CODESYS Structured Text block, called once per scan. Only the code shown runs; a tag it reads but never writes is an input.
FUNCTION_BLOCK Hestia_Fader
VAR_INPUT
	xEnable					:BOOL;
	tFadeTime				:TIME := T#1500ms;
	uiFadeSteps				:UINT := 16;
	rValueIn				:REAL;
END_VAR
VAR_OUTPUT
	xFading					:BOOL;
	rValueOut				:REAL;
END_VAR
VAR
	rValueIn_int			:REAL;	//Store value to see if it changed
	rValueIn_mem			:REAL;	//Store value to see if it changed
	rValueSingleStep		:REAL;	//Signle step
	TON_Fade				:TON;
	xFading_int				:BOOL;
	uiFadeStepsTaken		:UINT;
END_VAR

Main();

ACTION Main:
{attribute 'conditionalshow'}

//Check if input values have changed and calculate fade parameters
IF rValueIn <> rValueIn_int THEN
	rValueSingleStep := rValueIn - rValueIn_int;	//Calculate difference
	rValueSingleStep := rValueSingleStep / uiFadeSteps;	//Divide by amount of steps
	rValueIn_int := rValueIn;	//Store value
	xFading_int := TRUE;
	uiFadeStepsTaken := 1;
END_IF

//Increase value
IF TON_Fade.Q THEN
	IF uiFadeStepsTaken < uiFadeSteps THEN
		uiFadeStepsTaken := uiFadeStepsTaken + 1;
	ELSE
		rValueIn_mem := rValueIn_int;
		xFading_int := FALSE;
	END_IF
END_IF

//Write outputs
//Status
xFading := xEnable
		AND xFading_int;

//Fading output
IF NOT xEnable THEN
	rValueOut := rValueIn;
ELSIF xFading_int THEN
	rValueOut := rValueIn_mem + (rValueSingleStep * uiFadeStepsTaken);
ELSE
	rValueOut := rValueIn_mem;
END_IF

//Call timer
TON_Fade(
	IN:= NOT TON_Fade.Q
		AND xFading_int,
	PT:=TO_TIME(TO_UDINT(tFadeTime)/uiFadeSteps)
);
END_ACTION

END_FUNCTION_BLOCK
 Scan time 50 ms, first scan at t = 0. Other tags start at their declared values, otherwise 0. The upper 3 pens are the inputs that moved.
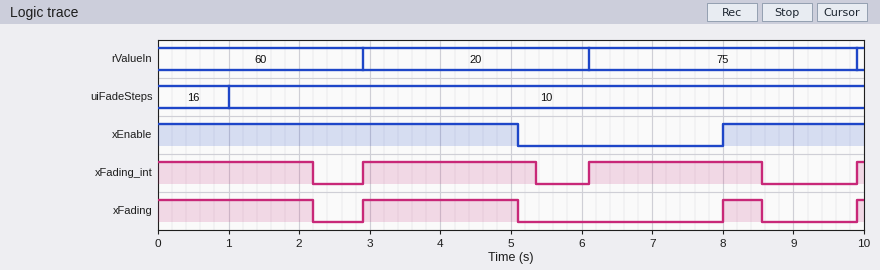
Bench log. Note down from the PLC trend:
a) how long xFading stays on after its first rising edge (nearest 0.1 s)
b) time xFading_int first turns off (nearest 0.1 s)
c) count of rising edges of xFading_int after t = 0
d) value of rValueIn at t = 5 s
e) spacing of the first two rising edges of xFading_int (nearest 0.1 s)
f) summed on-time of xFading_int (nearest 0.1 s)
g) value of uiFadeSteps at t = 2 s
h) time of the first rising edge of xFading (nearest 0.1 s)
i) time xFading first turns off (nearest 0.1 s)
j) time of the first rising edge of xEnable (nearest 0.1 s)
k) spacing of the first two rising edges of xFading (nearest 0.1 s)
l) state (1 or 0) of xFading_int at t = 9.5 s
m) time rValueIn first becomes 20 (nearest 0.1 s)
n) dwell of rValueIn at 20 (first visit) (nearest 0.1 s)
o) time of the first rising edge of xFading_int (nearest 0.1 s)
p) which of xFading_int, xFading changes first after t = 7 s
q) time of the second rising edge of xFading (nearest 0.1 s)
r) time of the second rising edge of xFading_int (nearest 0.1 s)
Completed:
2.2 s
2.2 s
3
20
3.2 s
7.2 s
10
2.9 s
2.2 s
8.0 s
5.1 s
0
2.9 s
3.2 s
2.9 s
xFading
8.0 s
6.1 s
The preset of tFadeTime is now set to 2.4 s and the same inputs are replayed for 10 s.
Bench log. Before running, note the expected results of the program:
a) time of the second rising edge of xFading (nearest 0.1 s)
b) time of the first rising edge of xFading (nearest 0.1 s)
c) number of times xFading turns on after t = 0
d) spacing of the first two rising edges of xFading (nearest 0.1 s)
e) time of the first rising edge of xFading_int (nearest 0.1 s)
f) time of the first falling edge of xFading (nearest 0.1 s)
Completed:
9.9 s
8.0 s
2
1.9 s
9.9 s
5.1 s
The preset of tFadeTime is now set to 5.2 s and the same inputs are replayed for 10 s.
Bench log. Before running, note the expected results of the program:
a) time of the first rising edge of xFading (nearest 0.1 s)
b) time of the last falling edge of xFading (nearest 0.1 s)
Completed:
8.0 s
5.1 s
